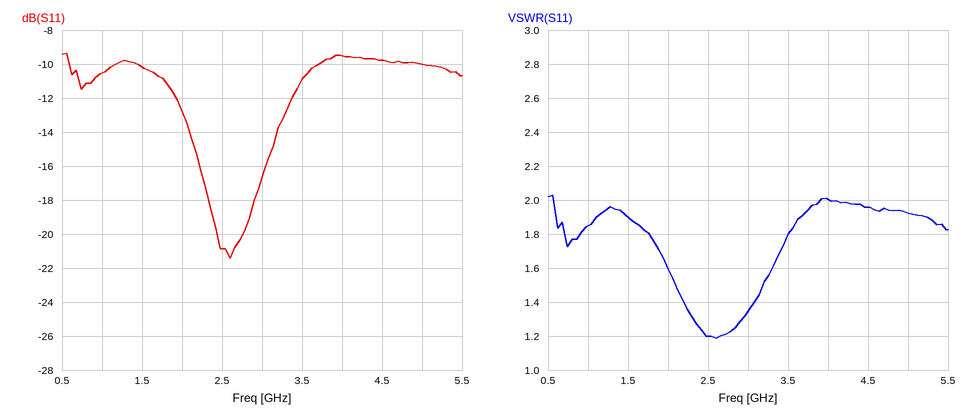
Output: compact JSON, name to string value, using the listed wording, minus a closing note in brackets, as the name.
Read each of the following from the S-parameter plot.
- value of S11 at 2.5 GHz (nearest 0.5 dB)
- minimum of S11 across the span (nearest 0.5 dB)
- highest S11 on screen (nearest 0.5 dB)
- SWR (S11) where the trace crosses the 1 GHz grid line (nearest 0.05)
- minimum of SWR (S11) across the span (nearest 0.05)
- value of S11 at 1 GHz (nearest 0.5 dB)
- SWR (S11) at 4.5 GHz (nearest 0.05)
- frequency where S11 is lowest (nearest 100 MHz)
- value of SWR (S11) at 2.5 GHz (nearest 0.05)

{"value of S11 at 2.5 GHz": "-21.0 dB", "minimum of S11 across the span": "-21.5 dB", "highest S11 on screen": "-9.5 dB", "SWR (S11) where the trace crosses the 1 GHz grid line": "1.85", "minimum of SWR (S11) across the span": "1.20", "value of S11 at 1 GHz": "-10.5 dB", "SWR (S11) at 4.5 GHz": "1.95", "frequency where S11 is lowest": "2.6 GHz", "value of SWR (S11) at 2.5 GHz": "1.20"}
